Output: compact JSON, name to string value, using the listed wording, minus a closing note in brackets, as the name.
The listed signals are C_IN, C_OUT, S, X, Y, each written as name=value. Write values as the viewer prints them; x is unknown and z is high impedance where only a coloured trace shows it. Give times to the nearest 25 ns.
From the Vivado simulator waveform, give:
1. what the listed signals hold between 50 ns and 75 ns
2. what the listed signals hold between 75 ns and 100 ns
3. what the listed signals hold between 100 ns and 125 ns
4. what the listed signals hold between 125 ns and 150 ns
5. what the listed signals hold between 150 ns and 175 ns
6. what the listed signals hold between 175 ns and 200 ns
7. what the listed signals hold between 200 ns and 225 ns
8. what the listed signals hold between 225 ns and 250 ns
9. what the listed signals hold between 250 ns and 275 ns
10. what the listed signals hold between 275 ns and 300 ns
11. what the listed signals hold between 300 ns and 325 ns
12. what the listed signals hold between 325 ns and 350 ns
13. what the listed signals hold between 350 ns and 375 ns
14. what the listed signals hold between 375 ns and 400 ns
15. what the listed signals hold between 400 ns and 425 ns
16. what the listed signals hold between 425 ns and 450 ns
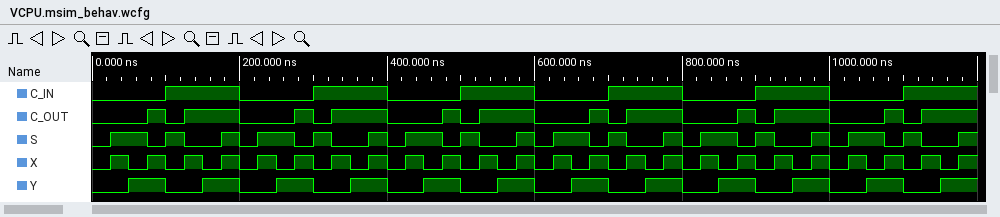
{"what the listed signals hold between 50 ns and 75 ns": "C_IN=0, C_OUT=0, S=1, X=0, Y=1", "what the listed signals hold between 75 ns and 100 ns": "C_IN=0, C_OUT=1, S=0, X=1, Y=1", "what the listed signals hold between 100 ns and 125 ns": "C_IN=1, C_OUT=0, S=1, X=0, Y=0", "what the listed signals hold between 125 ns and 150 ns": "C_IN=1, C_OUT=1, S=0, X=1, Y=0", "what the listed signals hold between 150 ns and 175 ns": "C_IN=1, C_OUT=1, S=0, X=0, Y=1", "what the listed signals hold between 175 ns and 200 ns": "C_IN=1, C_OUT=1, S=1, X=1, Y=1", "what the listed signals hold between 200 ns and 225 ns": "C_IN=0, C_OUT=0, S=0, X=0, Y=0", "what the listed signals hold between 225 ns and 250 ns": "C_IN=0, C_OUT=0, S=1, X=1, Y=0", "what the listed signals hold between 250 ns and 275 ns": "C_IN=0, C_OUT=0, S=1, X=0, Y=1", "what the listed signals hold between 275 ns and 300 ns": "C_IN=0, C_OUT=1, S=0, X=1, Y=1", "what the listed signals hold between 300 ns and 325 ns": "C_IN=1, C_OUT=0, S=1, X=0, Y=0", "what the listed signals hold between 325 ns and 350 ns": "C_IN=1, C_OUT=1, S=0, X=1, Y=0", "what the listed signals hold between 350 ns and 375 ns": "C_IN=1, C_OUT=1, S=0, X=0, Y=1", "what the listed signals hold between 375 ns and 400 ns": "C_IN=1, C_OUT=1, S=1, X=1, Y=1", "what the listed signals hold between 400 ns and 425 ns": "C_IN=0, C_OUT=0, S=0, X=0, Y=0", "what the listed signals hold between 425 ns and 450 ns": "C_IN=0, C_OUT=0, S=1, X=1, Y=0"}
